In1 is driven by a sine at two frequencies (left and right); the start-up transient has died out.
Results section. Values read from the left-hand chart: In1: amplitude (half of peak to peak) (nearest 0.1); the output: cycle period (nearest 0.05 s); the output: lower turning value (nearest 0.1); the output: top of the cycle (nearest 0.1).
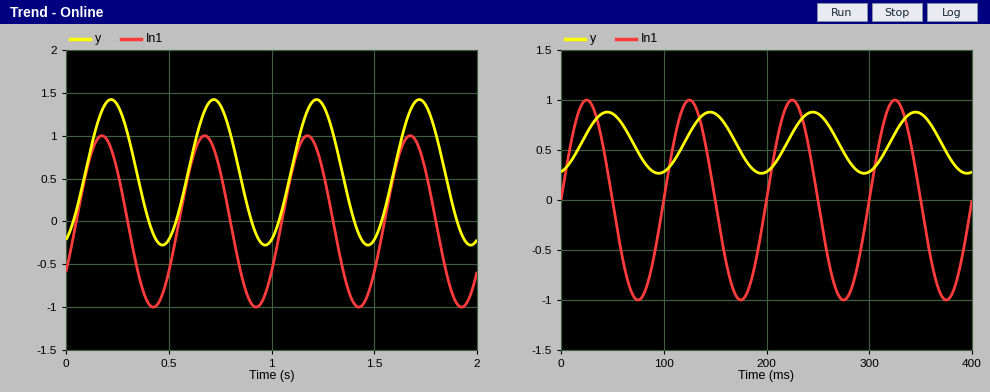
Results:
1.0
0.50 s
-0.3
1.4
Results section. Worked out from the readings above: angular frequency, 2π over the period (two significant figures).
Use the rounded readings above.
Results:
13 rad/s
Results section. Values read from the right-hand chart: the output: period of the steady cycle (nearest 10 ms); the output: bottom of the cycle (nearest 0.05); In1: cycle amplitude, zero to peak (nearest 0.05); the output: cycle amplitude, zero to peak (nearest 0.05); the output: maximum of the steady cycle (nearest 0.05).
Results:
100 ms
0.25
1.00
0.30
0.90
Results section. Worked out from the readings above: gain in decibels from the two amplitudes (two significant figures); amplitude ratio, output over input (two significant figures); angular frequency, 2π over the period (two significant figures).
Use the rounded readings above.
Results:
-10 dB
0.30
0.063 rad/ms
